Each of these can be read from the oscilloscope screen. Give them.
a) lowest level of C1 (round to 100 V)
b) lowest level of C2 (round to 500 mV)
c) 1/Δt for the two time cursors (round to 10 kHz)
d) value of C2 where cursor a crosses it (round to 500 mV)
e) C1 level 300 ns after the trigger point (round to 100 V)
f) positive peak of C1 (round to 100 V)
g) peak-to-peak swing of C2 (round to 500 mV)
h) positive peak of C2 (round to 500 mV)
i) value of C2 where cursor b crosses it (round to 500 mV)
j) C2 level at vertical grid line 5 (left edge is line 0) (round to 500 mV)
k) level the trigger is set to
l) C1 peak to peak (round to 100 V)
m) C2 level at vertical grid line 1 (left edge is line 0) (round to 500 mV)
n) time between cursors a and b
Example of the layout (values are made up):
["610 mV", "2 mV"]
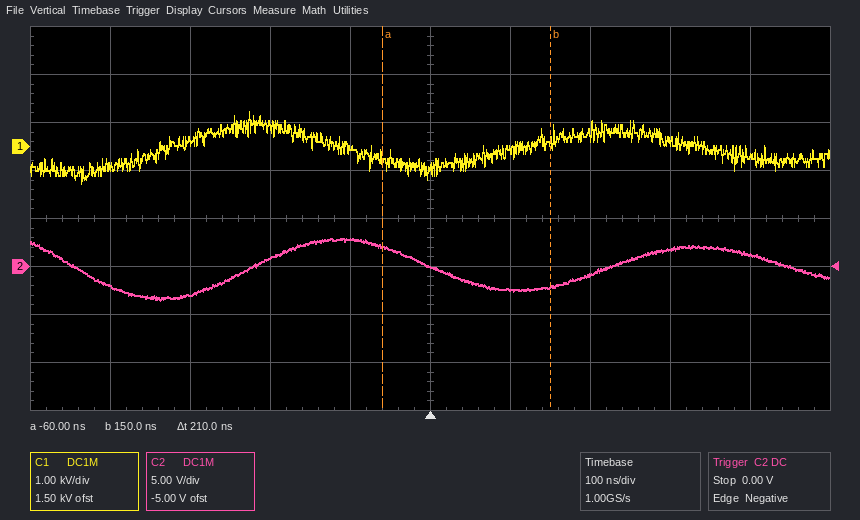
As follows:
["-800 V", "-3.5 V", "4.76 MHz", "2.0 V", "100 V", "700 V", "6.5 V", "3.0 V", "-2.0 V", "0.0 V", "0.00 V", "1.5 kV", "-2.0 V", "210 ns"]
